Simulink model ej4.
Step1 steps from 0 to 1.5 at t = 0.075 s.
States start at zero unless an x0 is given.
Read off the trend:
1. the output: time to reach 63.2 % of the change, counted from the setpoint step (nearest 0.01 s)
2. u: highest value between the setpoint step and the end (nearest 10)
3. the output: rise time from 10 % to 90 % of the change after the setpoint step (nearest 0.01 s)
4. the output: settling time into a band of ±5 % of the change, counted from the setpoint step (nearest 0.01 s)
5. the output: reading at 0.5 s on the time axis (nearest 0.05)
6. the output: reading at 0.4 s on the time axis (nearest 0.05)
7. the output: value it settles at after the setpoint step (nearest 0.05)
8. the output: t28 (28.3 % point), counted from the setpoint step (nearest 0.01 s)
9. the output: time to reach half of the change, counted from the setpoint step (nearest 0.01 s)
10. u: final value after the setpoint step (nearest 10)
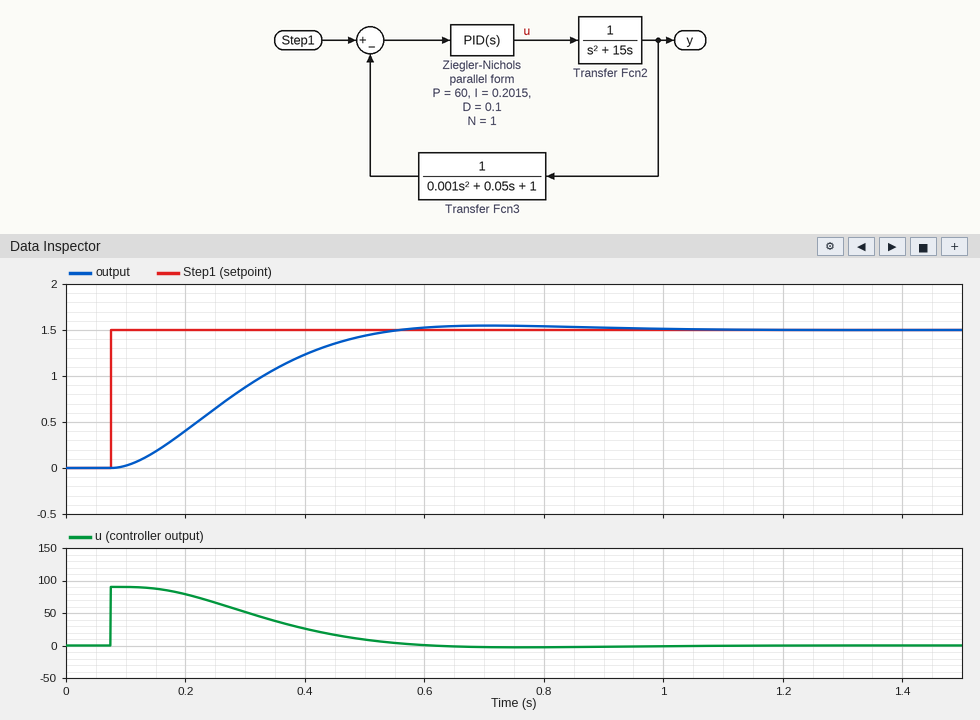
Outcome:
0.24 s
90
0.31 s
0.42 s
1.45
1.25
1.50
0.13 s
0.20 s
0
